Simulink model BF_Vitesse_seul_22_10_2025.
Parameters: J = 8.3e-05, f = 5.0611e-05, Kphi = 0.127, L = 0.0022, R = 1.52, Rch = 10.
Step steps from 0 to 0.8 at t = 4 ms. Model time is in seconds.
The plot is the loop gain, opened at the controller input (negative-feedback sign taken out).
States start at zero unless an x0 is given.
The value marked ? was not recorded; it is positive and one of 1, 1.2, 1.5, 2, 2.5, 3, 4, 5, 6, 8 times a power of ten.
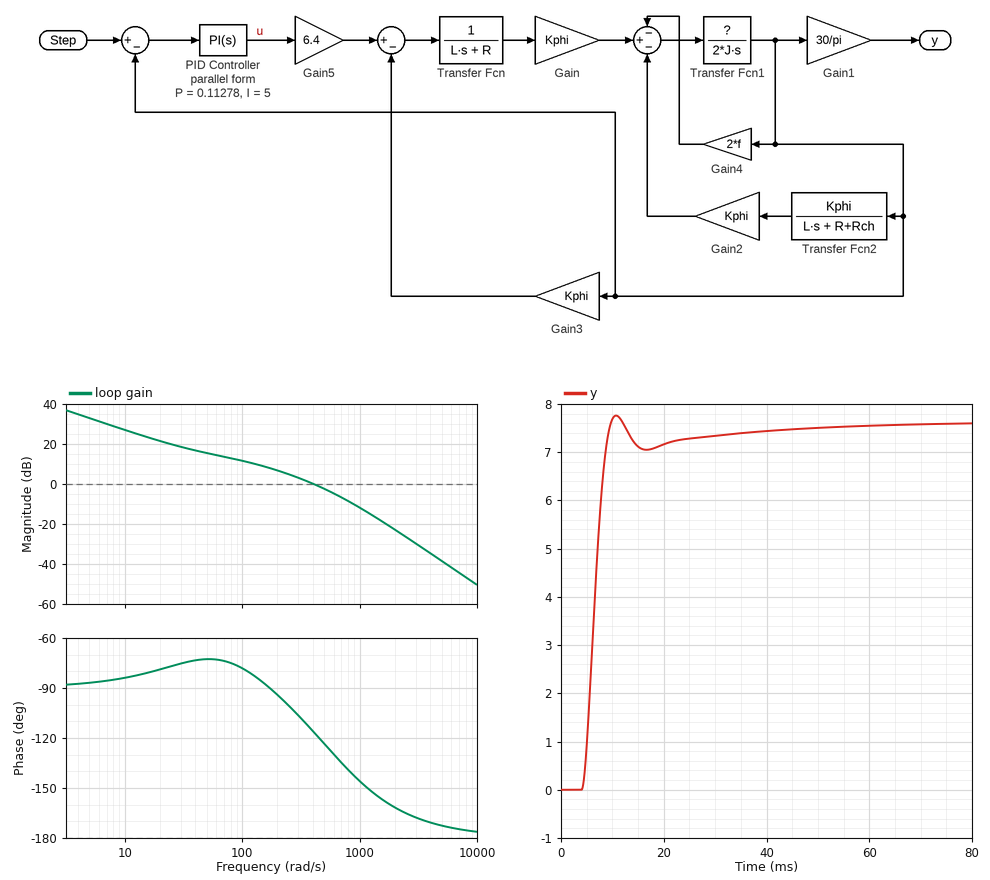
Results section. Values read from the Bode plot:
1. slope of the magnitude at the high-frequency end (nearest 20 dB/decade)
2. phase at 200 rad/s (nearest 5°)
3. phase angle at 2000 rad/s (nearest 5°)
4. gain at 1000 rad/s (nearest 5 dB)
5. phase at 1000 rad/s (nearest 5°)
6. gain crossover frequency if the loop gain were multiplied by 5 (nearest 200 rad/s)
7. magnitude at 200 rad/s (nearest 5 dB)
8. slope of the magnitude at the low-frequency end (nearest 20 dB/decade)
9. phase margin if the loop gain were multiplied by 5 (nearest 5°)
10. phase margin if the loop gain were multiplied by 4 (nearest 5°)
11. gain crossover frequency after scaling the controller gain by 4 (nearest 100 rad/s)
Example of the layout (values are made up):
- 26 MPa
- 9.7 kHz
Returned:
- -40 dB/decade
- -95°
- -160°
- -10 dB
- -145°
- 1200 rad/s
- 5 dB
- -20 dB/decade
- 30°
- 35°
- 1000 rad/s
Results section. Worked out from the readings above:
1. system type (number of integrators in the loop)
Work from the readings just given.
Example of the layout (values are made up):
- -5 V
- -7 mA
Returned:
- 1
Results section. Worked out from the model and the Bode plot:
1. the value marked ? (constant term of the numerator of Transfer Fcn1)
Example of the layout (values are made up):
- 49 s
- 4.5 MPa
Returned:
- 1.2
